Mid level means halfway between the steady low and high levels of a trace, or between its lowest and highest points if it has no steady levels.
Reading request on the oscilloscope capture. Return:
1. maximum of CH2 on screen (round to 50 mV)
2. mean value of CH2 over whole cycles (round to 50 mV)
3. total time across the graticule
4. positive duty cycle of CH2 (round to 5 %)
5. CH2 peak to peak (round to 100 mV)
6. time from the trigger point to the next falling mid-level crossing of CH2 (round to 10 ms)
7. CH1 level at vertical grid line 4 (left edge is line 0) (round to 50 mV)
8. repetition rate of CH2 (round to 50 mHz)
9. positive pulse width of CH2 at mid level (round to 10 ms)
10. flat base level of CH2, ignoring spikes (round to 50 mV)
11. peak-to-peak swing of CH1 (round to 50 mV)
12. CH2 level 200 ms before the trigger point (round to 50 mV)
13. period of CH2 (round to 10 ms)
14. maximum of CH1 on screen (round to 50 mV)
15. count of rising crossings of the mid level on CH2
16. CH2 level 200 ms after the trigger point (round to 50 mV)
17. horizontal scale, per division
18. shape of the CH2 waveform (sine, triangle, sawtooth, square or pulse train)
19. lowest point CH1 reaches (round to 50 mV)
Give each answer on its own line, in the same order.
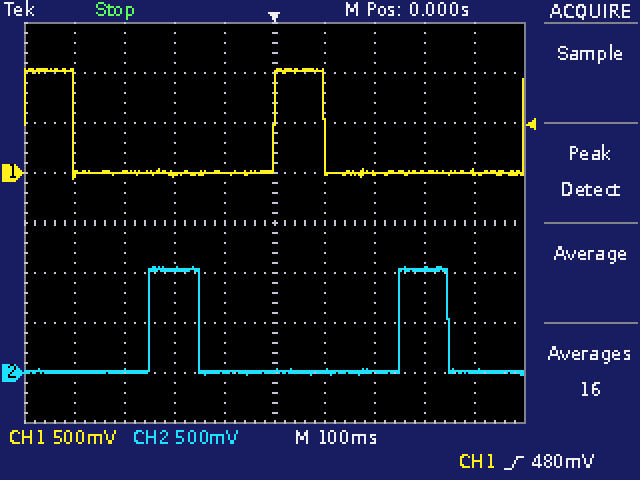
1.05 V
200 mV
1 s
20 %
1.10 V
350 ms
0 mV
2.00 Hz
100 ms
0 mV
1.10 V
1.05 V
500 ms
1.05 V
2
0 mV
100 ms
pulse train
-50 mV
